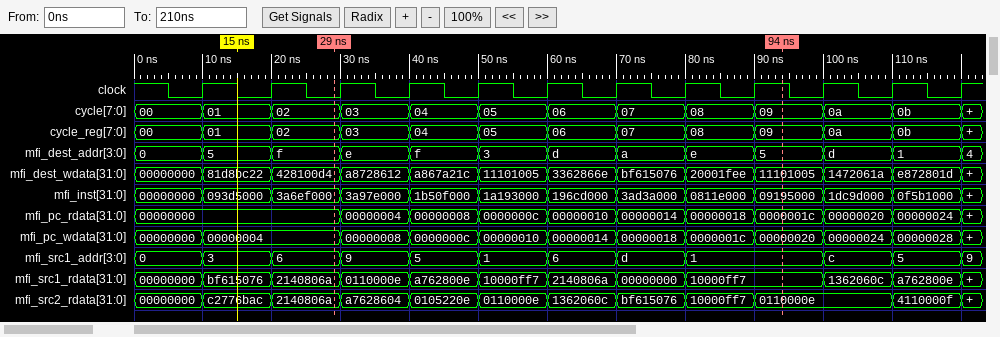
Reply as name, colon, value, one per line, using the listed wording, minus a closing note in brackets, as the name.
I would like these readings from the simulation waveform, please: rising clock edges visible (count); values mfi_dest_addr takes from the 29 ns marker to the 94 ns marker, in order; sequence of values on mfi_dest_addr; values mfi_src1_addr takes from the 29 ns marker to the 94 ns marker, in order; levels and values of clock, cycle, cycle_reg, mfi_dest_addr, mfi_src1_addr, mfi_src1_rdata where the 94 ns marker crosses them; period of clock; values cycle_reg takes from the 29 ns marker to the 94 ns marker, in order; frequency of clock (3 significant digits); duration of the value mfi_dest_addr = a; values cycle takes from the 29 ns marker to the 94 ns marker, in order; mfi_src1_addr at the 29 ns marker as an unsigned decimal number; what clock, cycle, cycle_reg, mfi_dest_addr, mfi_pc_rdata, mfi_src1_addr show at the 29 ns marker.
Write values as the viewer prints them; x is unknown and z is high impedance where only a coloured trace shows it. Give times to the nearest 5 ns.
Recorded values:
rising clock edges visible: 12
values mfi_dest_addr takes from the 29 ns marker to the 94 ns marker, in order: f, e, f, 3, d, a, e, 5
sequence of values on mfi_dest_addr: 0, 5, f, e, f, 3, d, a, e, 5, d, 1, 4
values mfi_src1_addr takes from the 29 ns marker to the 94 ns marker, in order: 6, 9, 5, 1, 6, d, 1
levels and values of clock, cycle, cycle_reg, mfi_dest_addr, mfi_src1_addr, mfi_src1_rdata where the 94 ns marker crosses them: clock=1, cycle=09, cycle_reg=09, mfi_dest_addr=5, mfi_src1_addr=1, mfi_src1_rdata=10000ff7
period of clock: 10 ns
values cycle_reg takes from the 29 ns marker to the 94 ns marker, in order: 02, 03, 04, 05, 06, 07, 08, 09
frequency of clock: 100 MHz
duration of the value mfi_dest_addr = a: 10 ns
values cycle takes from the 29 ns marker to the 94 ns marker, in order: 02, 03, 04, 05, 06, 07, 08, 09
mfi_src1_addr at the 29 ns marker as an unsigned decimal number: 6
what clock, cycle, cycle_reg, mfi_dest_addr, mfi_pc_rdata, mfi_src1_addr show at the 29 ns marker: clock=0, cycle=02, cycle_reg=02, mfi_dest_addr=f, mfi_pc_rdata=00000000, mfi_src1_addr=6
